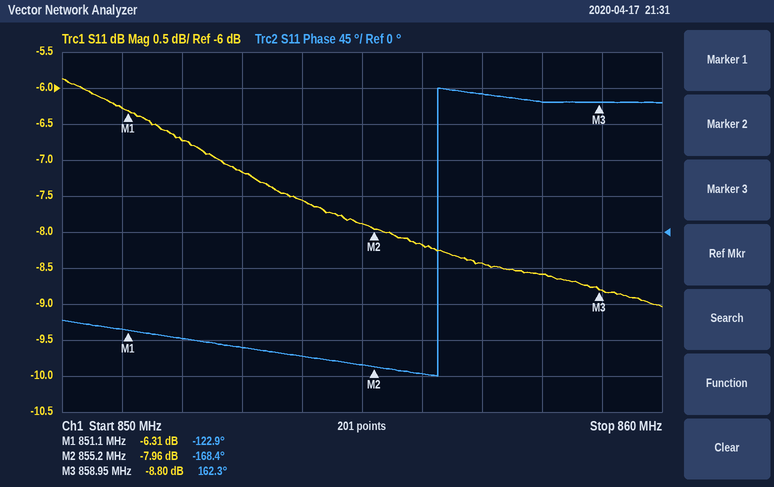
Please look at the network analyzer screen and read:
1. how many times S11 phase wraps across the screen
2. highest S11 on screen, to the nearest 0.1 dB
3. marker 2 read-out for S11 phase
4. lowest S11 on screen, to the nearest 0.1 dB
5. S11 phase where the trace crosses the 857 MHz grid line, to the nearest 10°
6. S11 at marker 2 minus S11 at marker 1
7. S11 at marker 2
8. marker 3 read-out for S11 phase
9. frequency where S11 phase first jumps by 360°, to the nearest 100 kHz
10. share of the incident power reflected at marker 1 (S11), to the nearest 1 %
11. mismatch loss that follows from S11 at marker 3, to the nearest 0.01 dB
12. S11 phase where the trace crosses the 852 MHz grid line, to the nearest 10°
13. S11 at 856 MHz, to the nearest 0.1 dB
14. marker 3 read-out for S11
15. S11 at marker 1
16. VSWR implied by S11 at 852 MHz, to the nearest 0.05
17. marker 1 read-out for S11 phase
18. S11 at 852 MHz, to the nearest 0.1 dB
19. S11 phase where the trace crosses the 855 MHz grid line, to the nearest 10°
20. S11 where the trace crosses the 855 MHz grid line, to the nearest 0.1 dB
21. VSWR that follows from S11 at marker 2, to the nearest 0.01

1
-5.9 dB
-168.4°
-9.0 dB
170°
-1.65 dB
-7.96 dB
162.3°
856.3 MHz
23 %
0.61 dB
-130°
-8.2 dB
-8.80 dB
-6.31 dB
2.70
-122.9°
-6.7 dB
-170°
-7.9 dB
2.33
